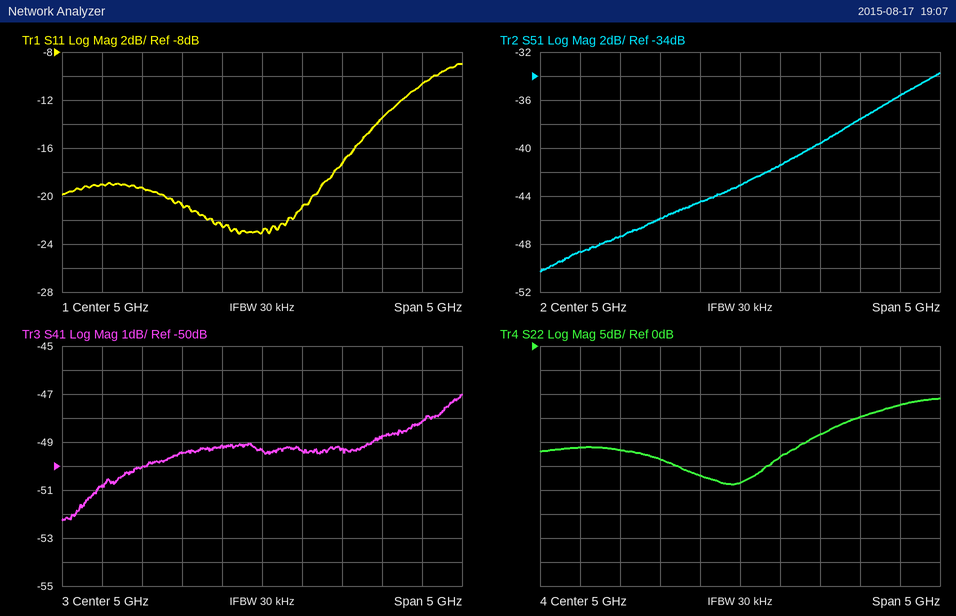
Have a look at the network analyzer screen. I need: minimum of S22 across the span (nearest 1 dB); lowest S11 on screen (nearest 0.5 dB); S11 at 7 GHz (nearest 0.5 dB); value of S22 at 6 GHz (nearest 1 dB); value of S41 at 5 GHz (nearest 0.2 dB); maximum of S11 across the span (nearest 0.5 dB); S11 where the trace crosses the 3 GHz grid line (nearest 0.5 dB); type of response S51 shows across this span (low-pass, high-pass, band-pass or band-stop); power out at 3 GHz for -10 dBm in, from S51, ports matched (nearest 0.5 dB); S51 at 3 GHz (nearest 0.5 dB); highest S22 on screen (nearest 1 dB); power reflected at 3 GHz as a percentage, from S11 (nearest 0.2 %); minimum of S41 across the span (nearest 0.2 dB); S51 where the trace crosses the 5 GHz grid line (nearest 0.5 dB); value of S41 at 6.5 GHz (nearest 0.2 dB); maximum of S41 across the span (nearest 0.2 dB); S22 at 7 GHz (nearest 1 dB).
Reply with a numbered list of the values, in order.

1. -29 dB
2. -23.0 dB
3. -10.5 dB
4. -18 dB
5. -49.4 dB
6. -9.0 dB
7. -19.0 dB
8. high-pass
9. -58.5 dBm
10. -48.5 dB
11. -11 dB
12. 1.2 %
13. -52.2 dB
14. -43.0 dB
15. -48.8 dB
16. -47.0 dB
17. -12 dB
